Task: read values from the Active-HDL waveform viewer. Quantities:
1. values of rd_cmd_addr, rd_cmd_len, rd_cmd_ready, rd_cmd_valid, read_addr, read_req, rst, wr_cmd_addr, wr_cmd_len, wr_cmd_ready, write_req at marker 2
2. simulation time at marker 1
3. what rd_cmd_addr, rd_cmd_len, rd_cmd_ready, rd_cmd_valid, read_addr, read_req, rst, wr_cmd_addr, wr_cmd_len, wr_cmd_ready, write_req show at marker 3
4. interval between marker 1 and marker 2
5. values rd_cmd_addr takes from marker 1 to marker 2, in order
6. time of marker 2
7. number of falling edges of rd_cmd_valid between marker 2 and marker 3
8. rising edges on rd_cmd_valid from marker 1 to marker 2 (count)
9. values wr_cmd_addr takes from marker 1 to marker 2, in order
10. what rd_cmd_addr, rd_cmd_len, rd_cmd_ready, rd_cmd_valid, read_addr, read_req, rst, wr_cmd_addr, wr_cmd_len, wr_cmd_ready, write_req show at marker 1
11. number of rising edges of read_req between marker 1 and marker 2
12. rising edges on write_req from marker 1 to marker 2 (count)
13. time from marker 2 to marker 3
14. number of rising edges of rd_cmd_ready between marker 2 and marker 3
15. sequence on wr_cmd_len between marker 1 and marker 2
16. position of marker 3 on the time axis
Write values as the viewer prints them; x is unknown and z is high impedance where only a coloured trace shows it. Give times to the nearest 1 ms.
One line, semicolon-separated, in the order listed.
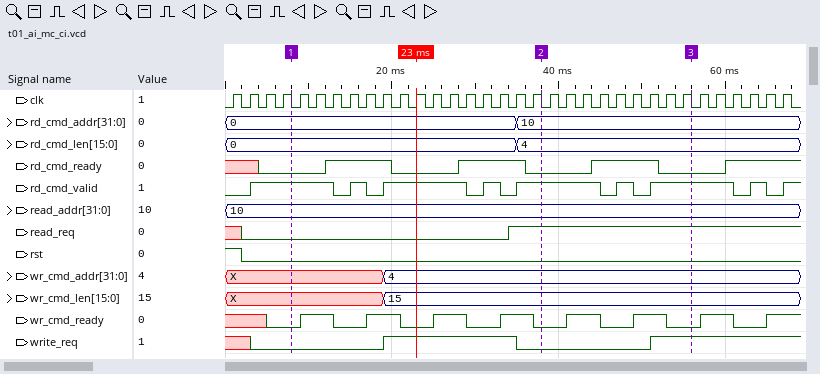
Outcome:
rd_cmd_addr=10, rd_cmd_len=4, rd_cmd_ready=0, rd_cmd_valid=1, read_addr=10, read_req=1, rst=0, wr_cmd_addr=4, wr_cmd_len=15, wr_cmd_ready=0, write_req=0; 8 ms; rd_cmd_addr=10, rd_cmd_len=4, rd_cmd_ready=0, rd_cmd_valid=1, read_addr=10, read_req=1, rst=0, wr_cmd_addr=4, wr_cmd_len=15, wr_cmd_ready=0, write_req=1; 30 ms; 0, 10; 38 ms; 2; 4; X, 4; rd_cmd_addr=0, rd_cmd_len=0, rd_cmd_ready=0, rd_cmd_valid=1, read_addr=10, read_req=0, rst=0, wr_cmd_addr=X, wr_cmd_len=X, wr_cmd_ready=0, write_req=0; 1; 1; 18 ms; 1; X, 15; 56 ms
